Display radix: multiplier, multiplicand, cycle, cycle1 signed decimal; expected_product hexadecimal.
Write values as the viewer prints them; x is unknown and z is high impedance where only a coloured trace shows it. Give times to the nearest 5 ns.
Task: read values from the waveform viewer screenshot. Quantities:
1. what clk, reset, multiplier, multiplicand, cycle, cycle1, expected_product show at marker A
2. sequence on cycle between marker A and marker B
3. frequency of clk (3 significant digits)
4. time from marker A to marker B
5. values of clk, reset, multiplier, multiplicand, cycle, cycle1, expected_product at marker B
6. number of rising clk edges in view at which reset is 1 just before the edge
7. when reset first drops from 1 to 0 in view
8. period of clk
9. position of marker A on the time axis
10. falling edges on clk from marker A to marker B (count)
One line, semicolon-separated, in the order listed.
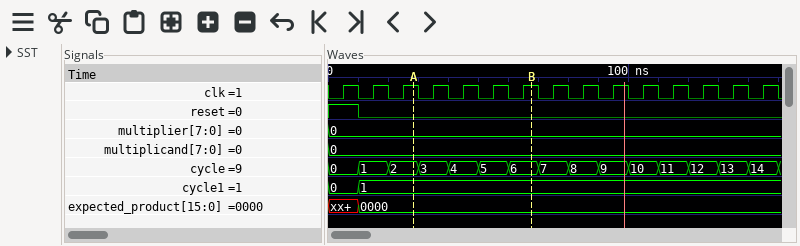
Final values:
clk=1, reset=0, multiplier=0, multiplicand=0, cycle=2, cycle1=1, expected_product=0000; 2, 3, 4, 5, 6; 100 MHz; 40 ns; clk=1, reset=0, multiplier=0, multiplicand=0, cycle=6, cycle1=1, expected_product=0000; 1; 10 ns; 10 ns; 30 ns; 4
